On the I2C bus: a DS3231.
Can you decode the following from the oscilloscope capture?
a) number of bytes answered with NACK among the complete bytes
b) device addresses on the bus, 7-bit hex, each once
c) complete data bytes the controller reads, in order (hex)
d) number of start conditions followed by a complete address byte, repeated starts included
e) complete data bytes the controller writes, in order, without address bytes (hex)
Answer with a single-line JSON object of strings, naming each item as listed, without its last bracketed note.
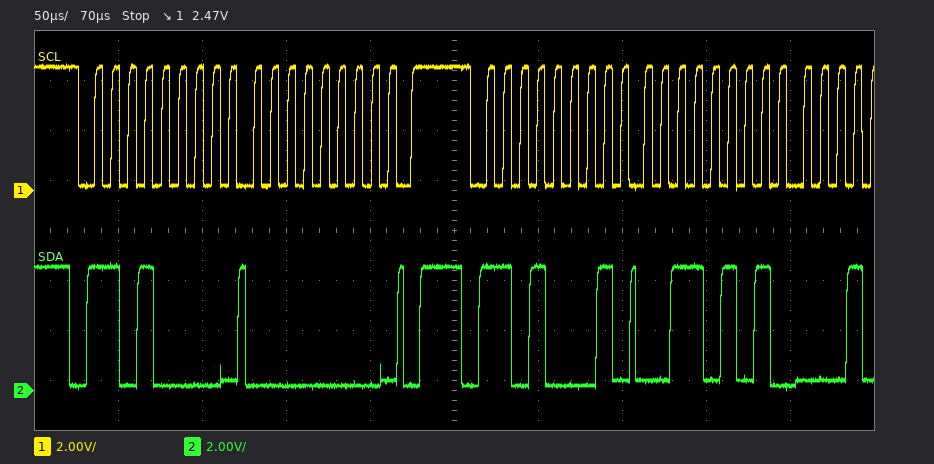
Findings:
{"number of bytes answered with NACK among the complete bytes": "0", "device addresses on the bus, 7-bit hex, each once": "0x68", "complete data bytes the controller reads, in order": "35", "number of start conditions followed by a complete address byte, repeated starts included": "2", "complete data bytes the controller writes, in order, without address bytes": "00"}
